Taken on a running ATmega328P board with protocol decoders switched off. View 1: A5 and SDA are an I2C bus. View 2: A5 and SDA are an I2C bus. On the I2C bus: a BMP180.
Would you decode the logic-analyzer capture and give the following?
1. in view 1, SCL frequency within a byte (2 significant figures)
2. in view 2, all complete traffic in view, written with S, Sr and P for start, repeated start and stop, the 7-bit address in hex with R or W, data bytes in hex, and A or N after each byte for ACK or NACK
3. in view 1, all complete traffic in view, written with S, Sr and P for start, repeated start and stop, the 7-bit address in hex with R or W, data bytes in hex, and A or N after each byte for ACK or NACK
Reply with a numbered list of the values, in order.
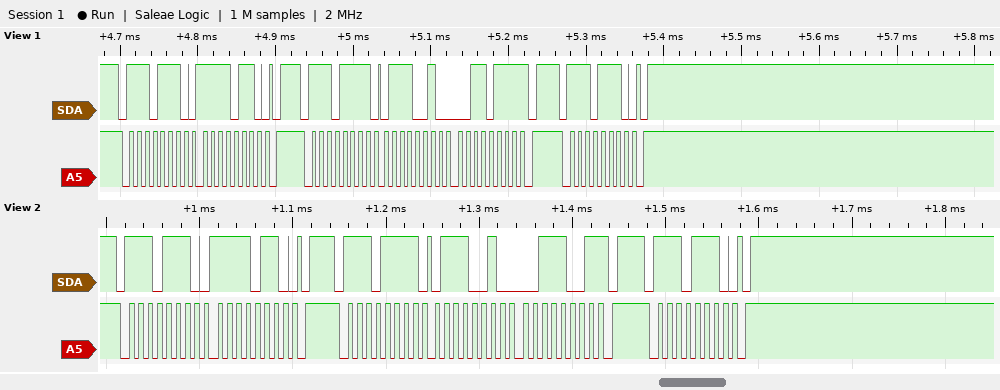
1. 100 kHz
2. S 77W A F6 A P S 77R A 72 A 39 N P S 77W A P
3. S 77W A F6 A P S 77R A 72 A 37 N P S 77W A P
